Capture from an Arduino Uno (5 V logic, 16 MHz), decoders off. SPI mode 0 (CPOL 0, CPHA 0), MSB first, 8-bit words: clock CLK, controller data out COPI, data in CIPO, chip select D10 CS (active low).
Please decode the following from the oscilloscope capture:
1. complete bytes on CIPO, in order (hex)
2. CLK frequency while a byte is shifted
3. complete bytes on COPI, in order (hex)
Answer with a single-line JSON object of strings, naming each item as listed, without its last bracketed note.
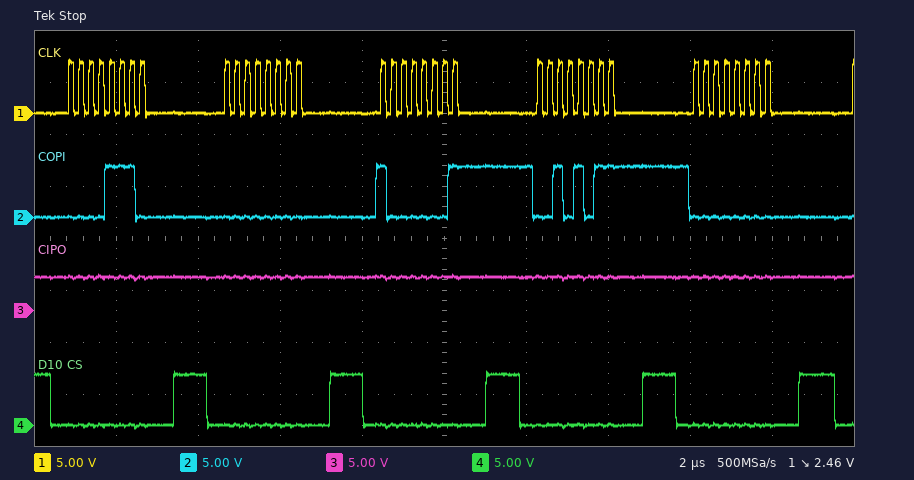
{"complete bytes on CIPO, in order": "0xFF 0xFF 0xFF 0xFF 0xFF", "CLK frequency while a byte is shifted": "4 MHz", "complete bytes on COPI, in order": "0x0E 0x00 0x81 0x2B 0x00"}
